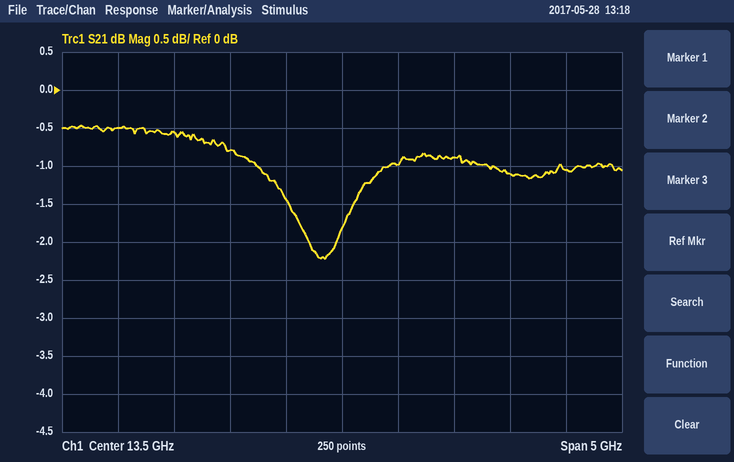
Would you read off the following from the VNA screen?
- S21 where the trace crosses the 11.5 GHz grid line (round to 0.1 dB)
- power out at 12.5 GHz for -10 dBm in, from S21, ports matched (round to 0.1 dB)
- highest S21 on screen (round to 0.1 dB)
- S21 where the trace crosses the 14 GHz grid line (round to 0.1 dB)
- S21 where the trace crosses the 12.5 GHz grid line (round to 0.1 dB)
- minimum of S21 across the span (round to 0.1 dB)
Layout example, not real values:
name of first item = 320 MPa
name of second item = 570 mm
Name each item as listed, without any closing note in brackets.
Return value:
S21 where the trace crosses the 11.5 GHz grid line = -0.5 dB
power out at 12.5 GHz for -10 dBm in, from S21, ports matched = -10.8 dBm
highest S21 on screen = -0.5 dB
S21 where the trace crosses the 14 GHz grid line = -1.0 dB
S21 where the trace crosses the 12.5 GHz grid line = -0.8 dB
minimum of S21 across the span = -2.2 dB
